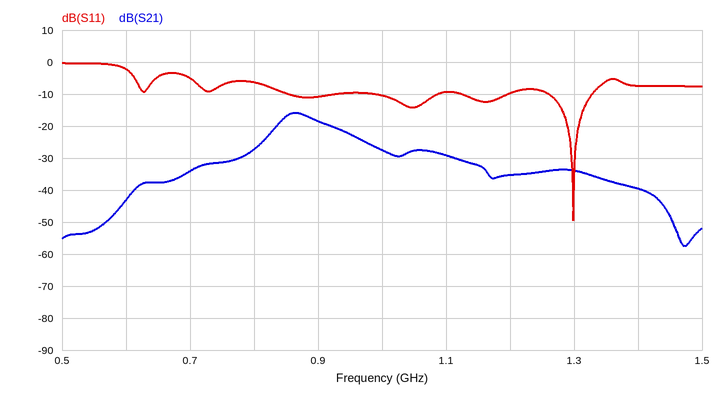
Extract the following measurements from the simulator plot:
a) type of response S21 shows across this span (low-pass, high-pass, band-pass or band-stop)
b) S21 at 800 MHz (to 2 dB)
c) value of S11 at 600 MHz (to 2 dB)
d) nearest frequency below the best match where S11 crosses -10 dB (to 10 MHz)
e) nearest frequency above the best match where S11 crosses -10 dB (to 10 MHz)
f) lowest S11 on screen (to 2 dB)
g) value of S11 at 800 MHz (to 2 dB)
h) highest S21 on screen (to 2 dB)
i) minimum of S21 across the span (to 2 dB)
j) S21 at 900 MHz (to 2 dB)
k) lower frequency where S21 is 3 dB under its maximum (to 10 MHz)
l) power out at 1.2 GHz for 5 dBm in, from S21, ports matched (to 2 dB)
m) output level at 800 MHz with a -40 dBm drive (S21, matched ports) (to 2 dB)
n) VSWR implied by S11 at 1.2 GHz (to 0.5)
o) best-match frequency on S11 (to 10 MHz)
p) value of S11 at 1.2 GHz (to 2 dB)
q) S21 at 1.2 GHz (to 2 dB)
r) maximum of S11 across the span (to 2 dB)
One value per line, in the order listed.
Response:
band-pass
-28 dB
-2 dB
1.26 GHz
1.33 GHz
-50 dB
-6 dB
-16 dB
-58 dB
-18 dB
840 MHz
-30 dBm
-68 dBm
2.0
1.30 GHz
-10 dB
-36 dB
0 dB
